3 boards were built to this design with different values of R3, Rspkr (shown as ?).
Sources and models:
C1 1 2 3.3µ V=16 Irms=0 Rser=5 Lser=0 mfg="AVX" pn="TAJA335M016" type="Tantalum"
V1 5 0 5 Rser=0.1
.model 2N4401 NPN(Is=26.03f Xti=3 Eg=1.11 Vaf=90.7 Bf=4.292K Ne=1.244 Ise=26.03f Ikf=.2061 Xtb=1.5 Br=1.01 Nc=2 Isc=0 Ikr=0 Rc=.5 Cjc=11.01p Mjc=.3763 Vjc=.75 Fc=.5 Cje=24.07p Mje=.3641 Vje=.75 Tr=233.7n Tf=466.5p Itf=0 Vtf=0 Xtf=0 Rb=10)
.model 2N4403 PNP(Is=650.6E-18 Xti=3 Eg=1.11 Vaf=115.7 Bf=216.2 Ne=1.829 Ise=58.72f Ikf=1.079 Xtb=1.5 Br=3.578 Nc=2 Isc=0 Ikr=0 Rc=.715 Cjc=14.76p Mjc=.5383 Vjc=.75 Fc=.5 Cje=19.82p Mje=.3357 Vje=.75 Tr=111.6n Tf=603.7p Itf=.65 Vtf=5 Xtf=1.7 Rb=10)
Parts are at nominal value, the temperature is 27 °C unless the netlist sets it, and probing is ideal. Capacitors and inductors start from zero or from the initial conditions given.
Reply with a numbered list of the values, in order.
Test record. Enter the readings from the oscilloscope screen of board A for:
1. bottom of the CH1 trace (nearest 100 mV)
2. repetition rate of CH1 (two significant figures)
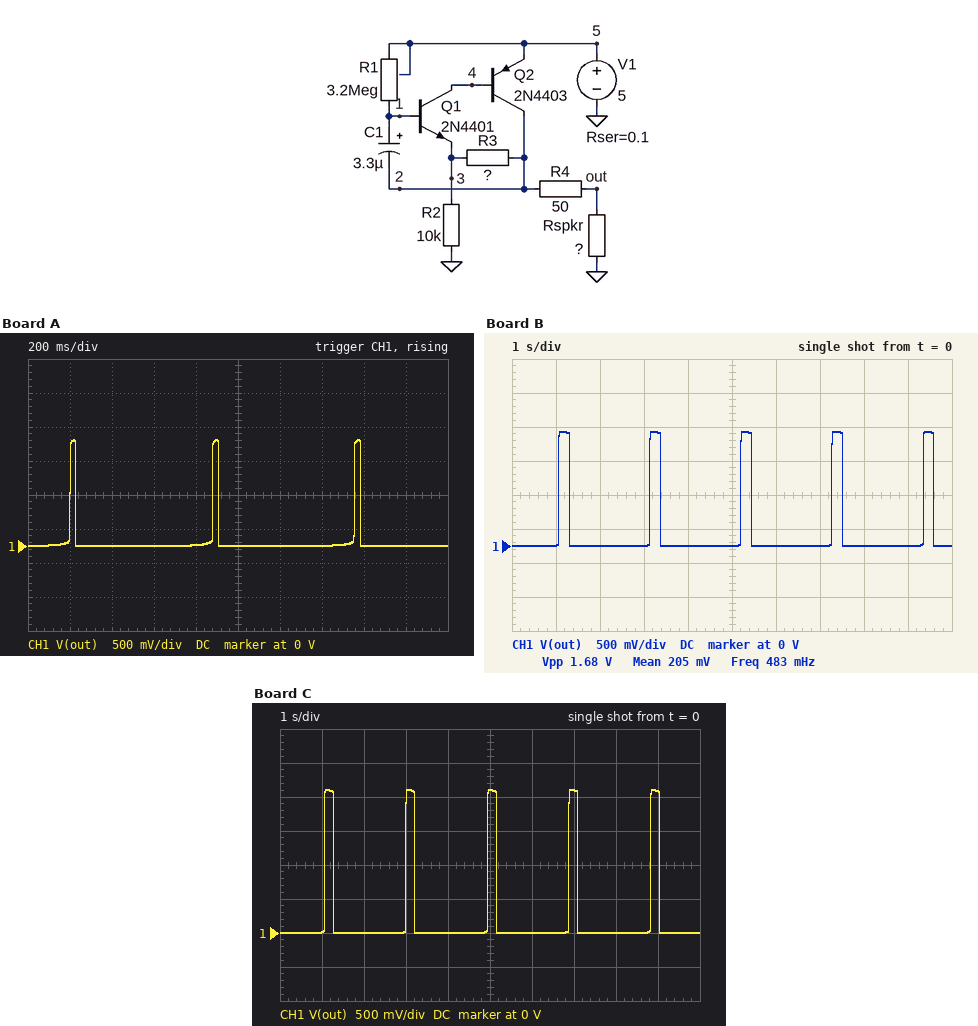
1. 0 V
2. 1.5 Hz
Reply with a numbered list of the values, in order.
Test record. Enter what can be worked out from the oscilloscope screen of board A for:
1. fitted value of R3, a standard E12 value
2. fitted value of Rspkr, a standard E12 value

1. 3.3 kΩ
2. 27 Ω
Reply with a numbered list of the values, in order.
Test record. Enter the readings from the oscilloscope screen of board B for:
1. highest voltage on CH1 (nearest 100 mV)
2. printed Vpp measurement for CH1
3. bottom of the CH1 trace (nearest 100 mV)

1. 1.7 V
2. 1.68 V
3. 0 V
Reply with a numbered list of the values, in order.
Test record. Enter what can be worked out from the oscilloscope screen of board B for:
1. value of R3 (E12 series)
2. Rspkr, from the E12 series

1. 15 kΩ
2. 27 Ω
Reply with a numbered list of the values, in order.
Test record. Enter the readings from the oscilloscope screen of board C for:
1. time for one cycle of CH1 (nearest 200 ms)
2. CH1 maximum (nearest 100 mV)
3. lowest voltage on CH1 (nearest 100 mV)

1. 2.0 s
2. 2.1 V
3. 0 V
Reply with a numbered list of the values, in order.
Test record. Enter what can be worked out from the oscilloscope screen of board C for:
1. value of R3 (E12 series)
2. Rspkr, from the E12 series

1. 8.2 kΩ
2. 39 Ω
